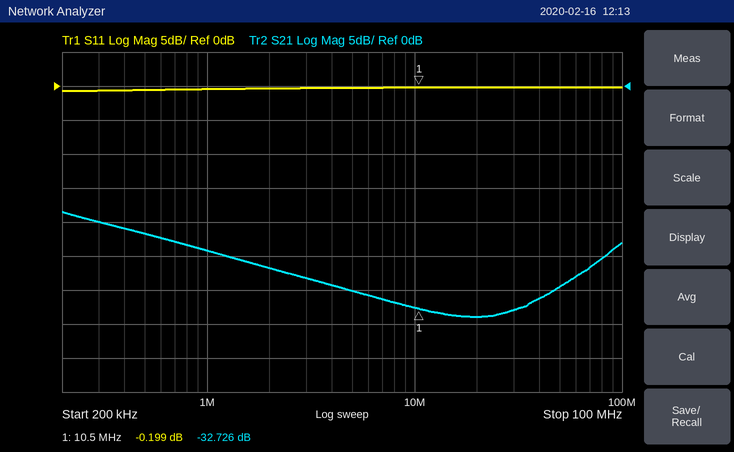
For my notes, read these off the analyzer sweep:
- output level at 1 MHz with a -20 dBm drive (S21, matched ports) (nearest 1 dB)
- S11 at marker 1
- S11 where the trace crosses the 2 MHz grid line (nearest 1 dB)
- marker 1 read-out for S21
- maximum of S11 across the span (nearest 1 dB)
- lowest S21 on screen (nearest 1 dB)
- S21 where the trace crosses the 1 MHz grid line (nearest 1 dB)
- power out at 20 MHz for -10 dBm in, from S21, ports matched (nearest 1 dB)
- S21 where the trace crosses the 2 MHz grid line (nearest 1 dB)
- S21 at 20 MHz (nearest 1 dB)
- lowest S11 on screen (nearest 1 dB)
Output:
-44 dBm
-0.199 dB
0 dB
-32.726 dB
0 dB
-34 dB
-24 dB
-44 dBm
-27 dB
-34 dB
-1 dB
